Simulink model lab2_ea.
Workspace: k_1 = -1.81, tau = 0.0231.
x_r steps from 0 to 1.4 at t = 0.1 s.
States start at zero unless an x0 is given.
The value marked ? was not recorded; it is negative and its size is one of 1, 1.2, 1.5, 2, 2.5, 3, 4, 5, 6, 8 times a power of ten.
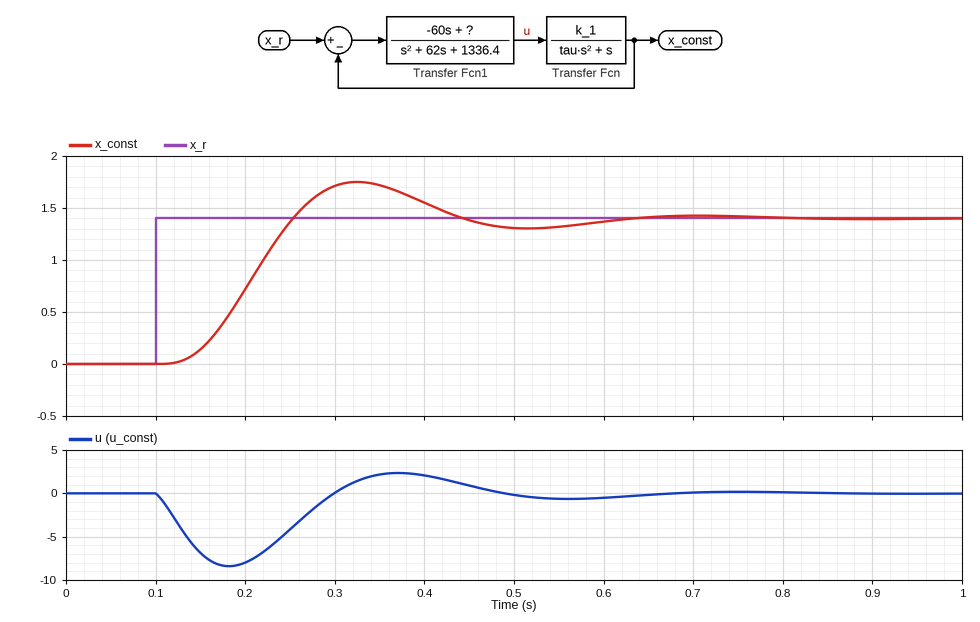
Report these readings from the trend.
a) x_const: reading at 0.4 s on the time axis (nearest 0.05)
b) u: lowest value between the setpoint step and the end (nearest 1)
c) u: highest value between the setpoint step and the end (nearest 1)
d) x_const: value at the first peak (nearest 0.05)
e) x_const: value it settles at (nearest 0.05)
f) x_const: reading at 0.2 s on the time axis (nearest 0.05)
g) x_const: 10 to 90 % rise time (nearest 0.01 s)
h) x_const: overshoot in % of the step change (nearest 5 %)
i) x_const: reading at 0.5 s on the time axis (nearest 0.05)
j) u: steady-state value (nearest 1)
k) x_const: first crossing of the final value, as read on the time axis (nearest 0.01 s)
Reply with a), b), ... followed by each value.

a) 1.55
b) -8
c) 2
d) 1.75
e) 1.40
f) 0.70
g) 0.09 s
h) 25 %
i) 1.30
j) 0
k) 0.25 s
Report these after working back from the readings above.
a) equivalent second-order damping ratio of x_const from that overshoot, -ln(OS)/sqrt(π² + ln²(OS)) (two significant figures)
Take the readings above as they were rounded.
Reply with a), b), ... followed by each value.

a) 0.40
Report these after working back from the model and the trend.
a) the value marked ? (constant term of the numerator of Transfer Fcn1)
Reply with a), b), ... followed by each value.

a) -10000
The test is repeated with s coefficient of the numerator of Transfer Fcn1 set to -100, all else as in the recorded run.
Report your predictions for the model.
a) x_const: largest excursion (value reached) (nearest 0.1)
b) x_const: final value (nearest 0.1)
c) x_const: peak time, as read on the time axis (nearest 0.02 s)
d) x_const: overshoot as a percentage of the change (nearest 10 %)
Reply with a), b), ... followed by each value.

a) 1.7
b) 1.4
c) 0.32 s
d) 20 %
